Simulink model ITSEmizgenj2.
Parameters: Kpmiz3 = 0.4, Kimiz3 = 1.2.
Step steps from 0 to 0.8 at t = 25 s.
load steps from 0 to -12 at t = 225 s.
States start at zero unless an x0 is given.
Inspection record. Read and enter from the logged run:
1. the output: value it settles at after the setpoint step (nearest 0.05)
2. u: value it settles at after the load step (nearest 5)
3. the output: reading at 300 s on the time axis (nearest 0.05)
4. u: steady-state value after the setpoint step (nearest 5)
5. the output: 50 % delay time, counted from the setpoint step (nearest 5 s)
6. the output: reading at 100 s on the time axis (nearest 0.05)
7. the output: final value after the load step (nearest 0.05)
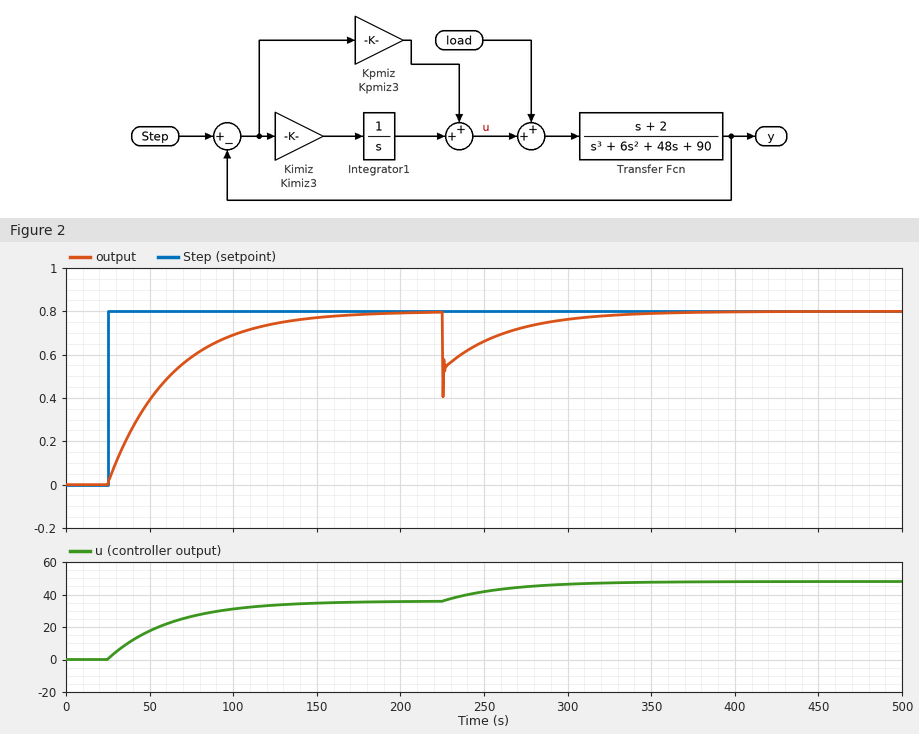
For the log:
0.80
50
0.75
35
25 s
0.70
0.80
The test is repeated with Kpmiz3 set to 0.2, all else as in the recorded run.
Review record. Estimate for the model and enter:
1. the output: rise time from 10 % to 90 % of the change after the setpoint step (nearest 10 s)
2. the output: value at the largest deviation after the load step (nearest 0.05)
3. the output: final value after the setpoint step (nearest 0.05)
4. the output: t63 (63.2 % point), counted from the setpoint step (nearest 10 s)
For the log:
80 s
0.40
0.80
40 s
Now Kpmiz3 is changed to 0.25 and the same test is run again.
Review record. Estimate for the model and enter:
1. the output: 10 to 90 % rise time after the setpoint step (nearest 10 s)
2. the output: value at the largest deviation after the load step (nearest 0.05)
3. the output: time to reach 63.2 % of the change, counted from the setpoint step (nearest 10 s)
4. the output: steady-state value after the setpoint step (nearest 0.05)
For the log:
80 s
0.40
40 s
0.80
